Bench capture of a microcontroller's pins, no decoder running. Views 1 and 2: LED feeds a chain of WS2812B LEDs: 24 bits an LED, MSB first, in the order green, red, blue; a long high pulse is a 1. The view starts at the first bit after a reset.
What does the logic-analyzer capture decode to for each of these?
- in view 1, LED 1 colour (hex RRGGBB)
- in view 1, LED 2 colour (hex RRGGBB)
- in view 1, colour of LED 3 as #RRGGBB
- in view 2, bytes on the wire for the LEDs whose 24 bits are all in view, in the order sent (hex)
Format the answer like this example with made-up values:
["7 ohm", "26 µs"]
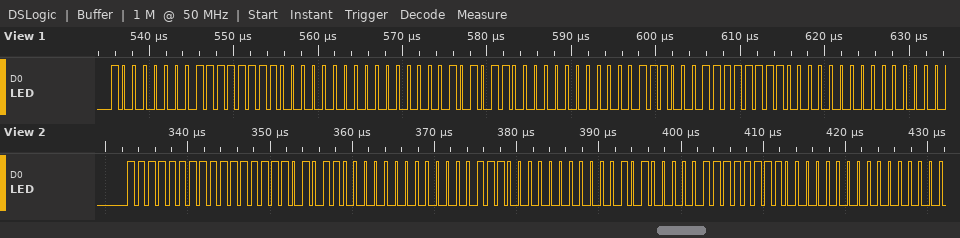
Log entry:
["#FF8000", "#AC0000", "#FF3800", "FF FF 58 00 38 00 A0 FF 00"]
